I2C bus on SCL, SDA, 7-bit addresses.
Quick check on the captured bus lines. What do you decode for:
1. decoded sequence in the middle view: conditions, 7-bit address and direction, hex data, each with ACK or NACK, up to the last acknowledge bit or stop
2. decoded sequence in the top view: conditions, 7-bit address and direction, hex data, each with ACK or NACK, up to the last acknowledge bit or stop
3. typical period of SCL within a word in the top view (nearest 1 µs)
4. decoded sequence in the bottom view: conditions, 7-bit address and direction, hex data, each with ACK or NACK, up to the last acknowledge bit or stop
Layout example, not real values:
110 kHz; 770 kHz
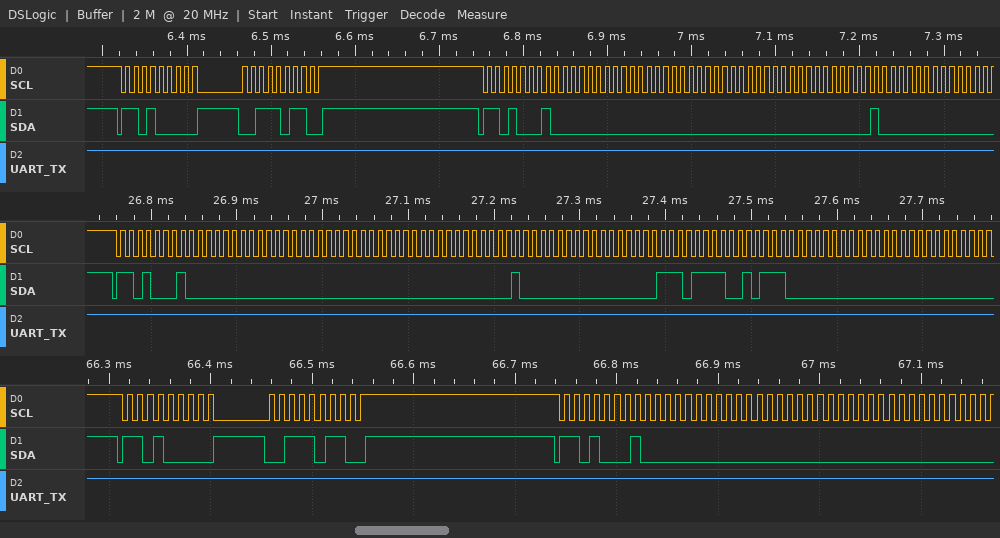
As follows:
start, address 68 read ACK, 00 ACK, 00 ACK, 00 ACK, 00 ACK, 40 ACK, 00 ACK, EF ACK, 5C ACK, 00 ACK, 00 ACK; start, address 68 write ACK, 3B ACK, stop, start, address 68 read ACK, 00 ACK, 00 ACK, 00 ACK, 00 ACK, 40 ACK; 10 µs; start, address 68 write ACK, 3B ACK, stop, start, address 68 read ACK, 00 ACK, 00 ACK, 00 ACK
